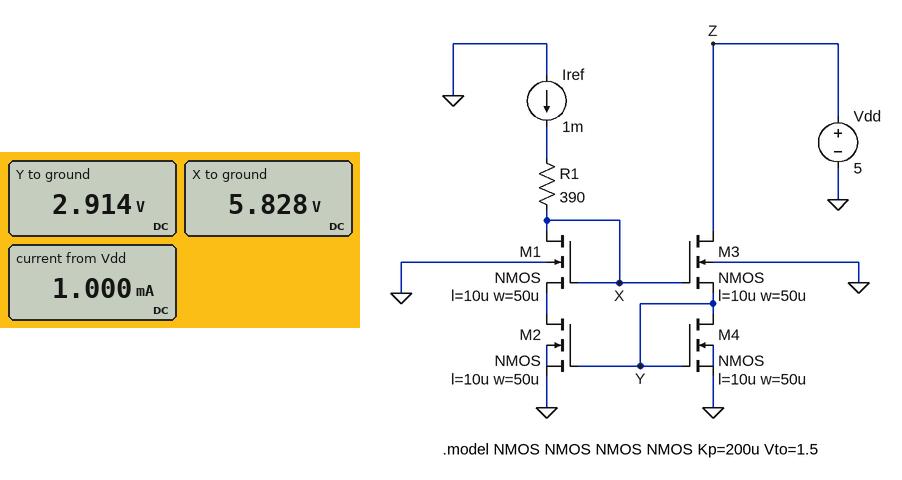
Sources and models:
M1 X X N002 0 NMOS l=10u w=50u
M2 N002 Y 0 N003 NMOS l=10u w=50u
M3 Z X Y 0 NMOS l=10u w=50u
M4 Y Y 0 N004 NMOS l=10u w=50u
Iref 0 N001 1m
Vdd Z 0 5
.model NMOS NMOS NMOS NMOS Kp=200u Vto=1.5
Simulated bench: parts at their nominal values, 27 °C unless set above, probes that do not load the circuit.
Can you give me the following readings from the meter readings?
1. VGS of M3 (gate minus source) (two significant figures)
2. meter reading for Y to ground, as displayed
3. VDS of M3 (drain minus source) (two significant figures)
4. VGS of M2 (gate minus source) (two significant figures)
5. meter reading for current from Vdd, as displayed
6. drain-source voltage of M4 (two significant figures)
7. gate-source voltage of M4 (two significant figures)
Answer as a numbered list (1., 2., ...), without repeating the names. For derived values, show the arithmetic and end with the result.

1. 5.828 V - 2.914 V = 2.9 V
2. 2.914 V
3. 5 V - 2.914 V = 2.1 V
4. 2.914 V = 2.9 V
5. 1.000 mA
6. 2.914 V = 2.9 V
7. 2.914 V = 2.9 V
